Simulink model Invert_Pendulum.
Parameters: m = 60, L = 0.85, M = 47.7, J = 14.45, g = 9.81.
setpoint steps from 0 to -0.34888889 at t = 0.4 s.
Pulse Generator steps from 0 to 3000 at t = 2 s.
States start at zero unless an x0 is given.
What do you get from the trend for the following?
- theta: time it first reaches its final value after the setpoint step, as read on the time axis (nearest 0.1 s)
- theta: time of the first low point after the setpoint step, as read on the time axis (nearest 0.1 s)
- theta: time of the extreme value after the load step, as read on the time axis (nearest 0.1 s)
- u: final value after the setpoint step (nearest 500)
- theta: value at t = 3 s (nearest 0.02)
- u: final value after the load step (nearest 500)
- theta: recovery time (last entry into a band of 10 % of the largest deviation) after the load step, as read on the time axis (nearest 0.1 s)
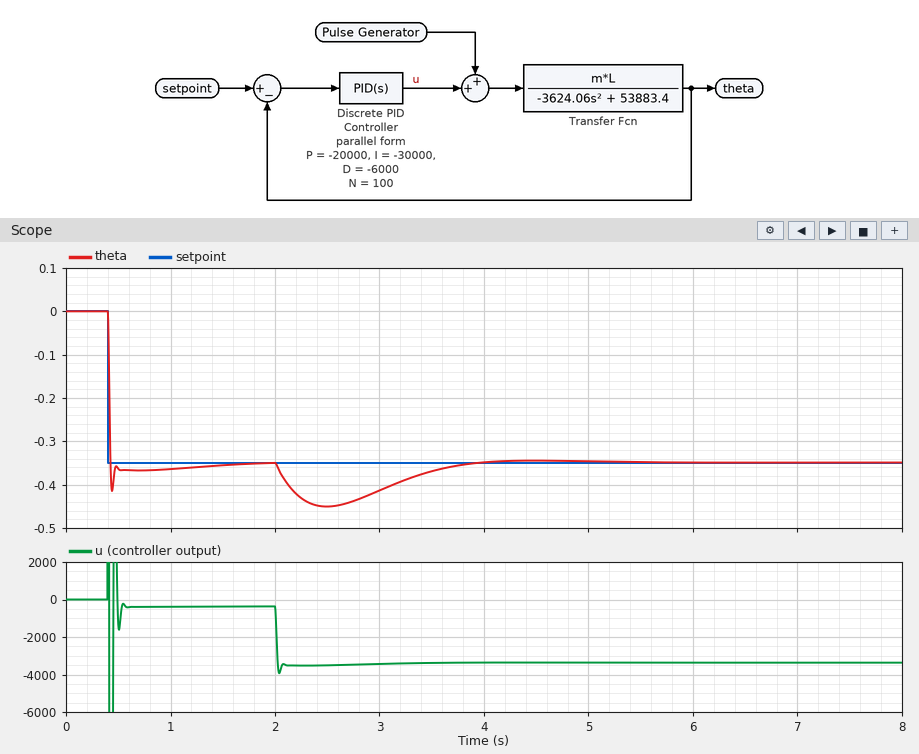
0.4 s
0.4 s
2.5 s
-500
-0.42
-3500
3.7 s
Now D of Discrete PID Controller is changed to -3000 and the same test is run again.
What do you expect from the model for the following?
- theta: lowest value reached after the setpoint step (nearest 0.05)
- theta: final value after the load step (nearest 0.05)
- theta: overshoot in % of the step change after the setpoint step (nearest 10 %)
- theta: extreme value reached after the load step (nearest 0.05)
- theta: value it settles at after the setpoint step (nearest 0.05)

-0.40
-0.35
20 %
-0.45
-0.35
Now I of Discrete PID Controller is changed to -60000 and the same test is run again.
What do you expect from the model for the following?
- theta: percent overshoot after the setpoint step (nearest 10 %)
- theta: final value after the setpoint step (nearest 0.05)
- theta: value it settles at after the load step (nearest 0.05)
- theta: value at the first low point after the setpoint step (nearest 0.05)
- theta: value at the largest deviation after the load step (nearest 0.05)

20 %
-0.35
-0.35
-0.40
-0.45
